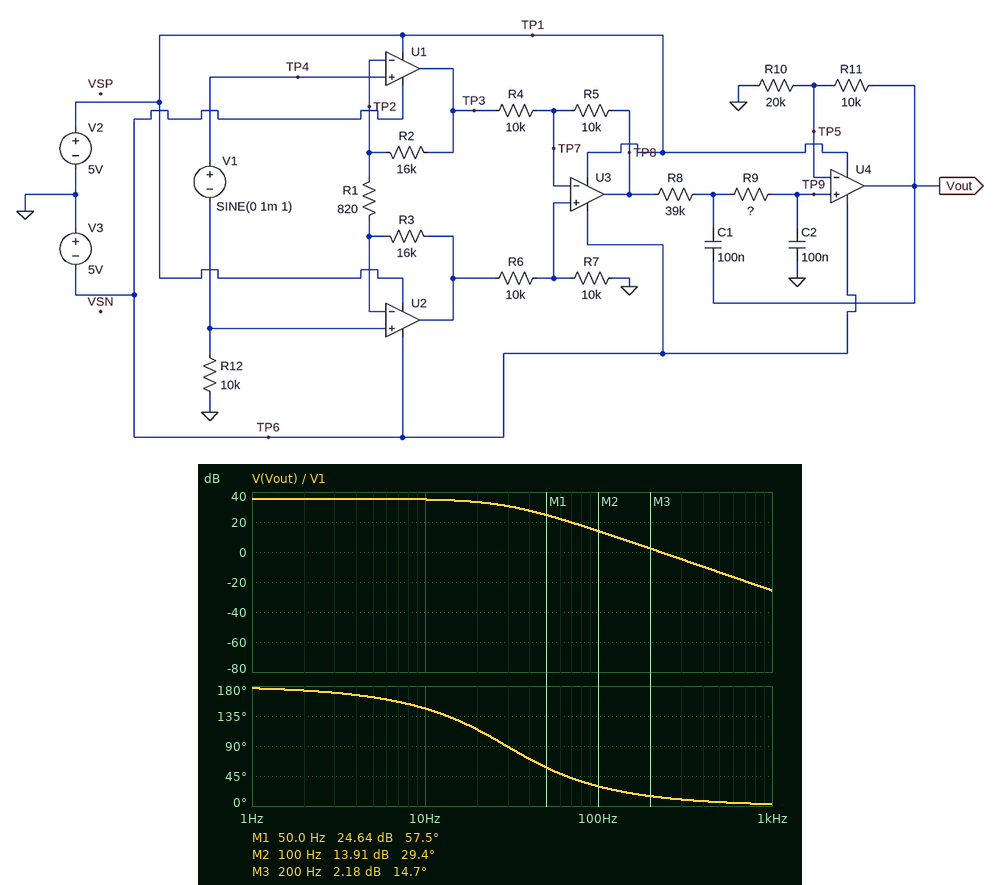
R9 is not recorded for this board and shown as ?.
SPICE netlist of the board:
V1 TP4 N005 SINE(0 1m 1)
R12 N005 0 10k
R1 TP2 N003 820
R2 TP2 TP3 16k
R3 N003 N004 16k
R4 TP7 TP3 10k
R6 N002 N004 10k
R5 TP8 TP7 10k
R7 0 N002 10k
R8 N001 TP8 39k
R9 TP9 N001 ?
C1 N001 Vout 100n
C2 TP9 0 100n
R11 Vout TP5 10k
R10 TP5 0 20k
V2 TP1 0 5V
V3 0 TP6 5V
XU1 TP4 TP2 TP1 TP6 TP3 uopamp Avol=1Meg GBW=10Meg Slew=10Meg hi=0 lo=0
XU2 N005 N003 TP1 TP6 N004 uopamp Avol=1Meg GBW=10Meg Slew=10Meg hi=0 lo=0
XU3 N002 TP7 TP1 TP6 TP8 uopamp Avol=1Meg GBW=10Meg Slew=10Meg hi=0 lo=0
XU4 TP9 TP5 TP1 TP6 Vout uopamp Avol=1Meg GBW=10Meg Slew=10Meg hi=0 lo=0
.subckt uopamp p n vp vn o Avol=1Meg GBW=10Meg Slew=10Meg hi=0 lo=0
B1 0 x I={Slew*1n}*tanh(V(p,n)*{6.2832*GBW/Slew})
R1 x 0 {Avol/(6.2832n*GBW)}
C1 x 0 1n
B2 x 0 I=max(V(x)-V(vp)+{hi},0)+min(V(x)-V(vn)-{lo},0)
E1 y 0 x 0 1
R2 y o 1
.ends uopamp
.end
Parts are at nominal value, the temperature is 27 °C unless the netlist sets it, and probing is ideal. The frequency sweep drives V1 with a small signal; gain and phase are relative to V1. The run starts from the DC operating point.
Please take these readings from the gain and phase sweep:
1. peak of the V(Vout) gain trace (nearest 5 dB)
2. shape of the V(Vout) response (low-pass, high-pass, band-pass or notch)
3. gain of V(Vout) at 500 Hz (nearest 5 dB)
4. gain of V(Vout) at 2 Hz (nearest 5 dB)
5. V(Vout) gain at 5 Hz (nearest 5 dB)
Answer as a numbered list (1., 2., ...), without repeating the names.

1. 35 dB
2. low-pass
3. -15 dB
4. 35 dB
5. 35 dB
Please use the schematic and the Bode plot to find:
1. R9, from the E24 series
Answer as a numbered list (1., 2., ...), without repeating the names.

1. 75 kΩ
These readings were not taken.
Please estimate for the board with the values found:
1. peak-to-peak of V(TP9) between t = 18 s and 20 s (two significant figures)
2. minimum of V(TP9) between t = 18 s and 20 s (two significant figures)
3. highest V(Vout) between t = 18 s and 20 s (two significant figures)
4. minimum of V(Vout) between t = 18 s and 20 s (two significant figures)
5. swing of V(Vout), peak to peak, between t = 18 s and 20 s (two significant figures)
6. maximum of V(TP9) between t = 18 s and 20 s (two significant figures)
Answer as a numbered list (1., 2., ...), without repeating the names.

1. 80 mV
2. -40 mV
3. 60 mV
4. -60 mV
5. 120 mV
6. 40 mV
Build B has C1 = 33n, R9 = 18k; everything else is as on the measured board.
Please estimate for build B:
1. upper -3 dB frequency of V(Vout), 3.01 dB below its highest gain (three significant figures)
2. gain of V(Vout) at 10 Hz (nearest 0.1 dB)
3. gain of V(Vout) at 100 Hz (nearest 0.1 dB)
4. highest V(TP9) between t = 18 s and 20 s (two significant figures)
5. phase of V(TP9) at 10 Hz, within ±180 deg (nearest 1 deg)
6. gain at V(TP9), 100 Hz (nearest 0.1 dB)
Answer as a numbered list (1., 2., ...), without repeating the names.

1. 34.6 Hz
2. 35.2 dB
3. 25.5 dB
4. 40 mV
5. 162 deg
6. 22.0 dB
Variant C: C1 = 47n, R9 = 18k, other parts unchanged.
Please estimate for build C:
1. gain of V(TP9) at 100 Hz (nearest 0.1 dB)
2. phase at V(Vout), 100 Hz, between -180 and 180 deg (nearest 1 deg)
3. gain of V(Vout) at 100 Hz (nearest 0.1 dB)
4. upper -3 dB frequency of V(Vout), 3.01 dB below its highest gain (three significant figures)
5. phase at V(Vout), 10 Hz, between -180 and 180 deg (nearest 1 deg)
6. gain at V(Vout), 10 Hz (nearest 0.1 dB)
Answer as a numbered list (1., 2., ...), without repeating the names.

1. 22.4 dB
2. 84 deg
3. 26.0 dB
4. 38.7 Hz
5. 163 deg
6. 35.3 dB
